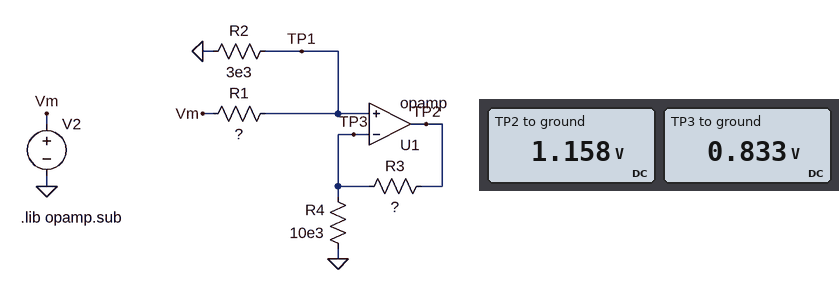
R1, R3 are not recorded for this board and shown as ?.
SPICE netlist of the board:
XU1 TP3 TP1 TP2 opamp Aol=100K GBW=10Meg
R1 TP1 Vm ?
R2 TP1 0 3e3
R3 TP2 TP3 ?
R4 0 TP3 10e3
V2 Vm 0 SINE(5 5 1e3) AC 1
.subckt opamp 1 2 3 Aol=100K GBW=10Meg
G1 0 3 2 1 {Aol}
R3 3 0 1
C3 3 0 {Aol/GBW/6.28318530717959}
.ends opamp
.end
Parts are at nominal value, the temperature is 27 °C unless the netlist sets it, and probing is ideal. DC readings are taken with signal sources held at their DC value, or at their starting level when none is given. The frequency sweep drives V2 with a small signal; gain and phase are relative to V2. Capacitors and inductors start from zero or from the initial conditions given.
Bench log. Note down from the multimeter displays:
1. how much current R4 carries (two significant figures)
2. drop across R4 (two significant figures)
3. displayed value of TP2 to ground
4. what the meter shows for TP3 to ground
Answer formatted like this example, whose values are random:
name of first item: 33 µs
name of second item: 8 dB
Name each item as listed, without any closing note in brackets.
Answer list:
how much current R4 carries: 83 µA
drop across R4: 830 mV
displayed value of TP2 to ground: 1.158 V
what the meter shows for TP3 to ground: 0.833 V
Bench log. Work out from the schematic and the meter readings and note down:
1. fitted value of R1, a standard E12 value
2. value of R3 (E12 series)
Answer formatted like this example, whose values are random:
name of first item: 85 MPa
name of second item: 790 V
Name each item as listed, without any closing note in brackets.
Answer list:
fitted value of R1, a standard E12 value: 15 kΩ
value of R3: 3.9 kΩ
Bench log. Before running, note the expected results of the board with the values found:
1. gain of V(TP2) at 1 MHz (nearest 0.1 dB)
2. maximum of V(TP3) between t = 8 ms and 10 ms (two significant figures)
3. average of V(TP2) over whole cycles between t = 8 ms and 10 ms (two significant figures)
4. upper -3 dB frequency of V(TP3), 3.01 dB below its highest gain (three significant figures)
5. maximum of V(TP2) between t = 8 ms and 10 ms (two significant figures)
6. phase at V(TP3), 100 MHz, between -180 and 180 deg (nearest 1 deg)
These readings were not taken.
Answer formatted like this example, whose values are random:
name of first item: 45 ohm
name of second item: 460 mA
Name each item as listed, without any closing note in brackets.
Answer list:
gain of V(TP2) at 1 MHz: -12.8 dB
maximum of V(TP3) between t = 8 ms and 10 ms: 1.7 V
average of V(TP2) over whole cycles between t = 8 ms and 10 ms: 1.2 V
upper -3 dB frequency of V(TP3), 3.01 dB below its highest gain: 7.19 MHz
maximum of V(TP2) between t = 8 ms and 10 ms: 2.3 V
phase at V(TP3), 100 MHz, between -180 and 180 deg: -86 deg
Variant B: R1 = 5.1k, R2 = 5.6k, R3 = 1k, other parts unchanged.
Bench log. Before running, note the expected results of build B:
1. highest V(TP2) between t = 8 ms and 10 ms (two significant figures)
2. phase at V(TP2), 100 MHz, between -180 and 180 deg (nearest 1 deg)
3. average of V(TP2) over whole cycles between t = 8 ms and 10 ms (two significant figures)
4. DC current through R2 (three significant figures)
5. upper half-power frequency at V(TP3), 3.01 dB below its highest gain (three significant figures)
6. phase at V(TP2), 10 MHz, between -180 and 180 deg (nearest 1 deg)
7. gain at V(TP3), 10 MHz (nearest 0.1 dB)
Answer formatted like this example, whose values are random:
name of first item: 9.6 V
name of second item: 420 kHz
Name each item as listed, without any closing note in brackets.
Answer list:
highest V(TP2) between t = 8 ms and 10 ms: 5.8 V
phase at V(TP2), 100 MHz, between -180 and 180 deg: -85 deg
average of V(TP2) over whole cycles between t = 8 ms and 10 ms: 2.9 V
DC current through R2: 467 µA
upper half-power frequency at V(TP3), 3.01 dB below its highest gain: 9.09 MHz
phase at V(TP2), 10 MHz, between -180 and 180 deg: -48 deg
gain at V(TP3), 10 MHz: -9.1 dB
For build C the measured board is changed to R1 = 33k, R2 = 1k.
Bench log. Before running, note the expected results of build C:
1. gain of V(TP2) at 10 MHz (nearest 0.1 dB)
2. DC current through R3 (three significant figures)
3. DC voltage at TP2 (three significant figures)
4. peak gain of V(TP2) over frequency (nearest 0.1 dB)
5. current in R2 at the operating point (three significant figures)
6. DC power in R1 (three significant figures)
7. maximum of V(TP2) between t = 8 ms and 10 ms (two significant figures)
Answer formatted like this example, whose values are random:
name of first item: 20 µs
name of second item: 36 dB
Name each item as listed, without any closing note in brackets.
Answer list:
gain of V(TP2) at 10 MHz: -32.4 dB
DC current through R3: 14.7 µA
DC voltage at TP2: 204 mV
peak gain of V(TP2) over frequency: -27.8 dB
current in R2 at the operating point: 147 µA
DC power in R1: 714 µW
maximum of V(TP2) between t = 8 ms and 10 ms: 410 mV
